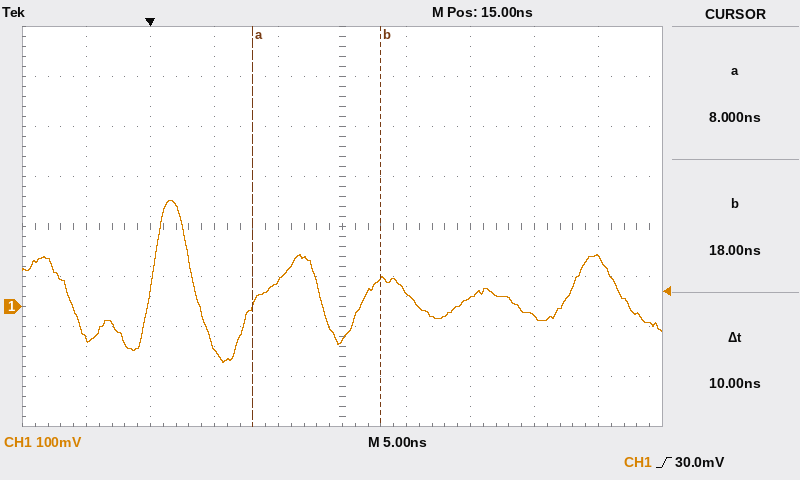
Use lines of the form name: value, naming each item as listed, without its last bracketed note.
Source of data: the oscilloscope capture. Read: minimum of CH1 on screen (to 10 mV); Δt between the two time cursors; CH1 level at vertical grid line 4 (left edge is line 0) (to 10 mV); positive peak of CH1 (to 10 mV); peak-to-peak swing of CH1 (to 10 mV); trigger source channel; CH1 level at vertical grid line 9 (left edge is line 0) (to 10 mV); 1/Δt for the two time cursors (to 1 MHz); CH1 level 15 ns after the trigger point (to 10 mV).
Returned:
minimum of CH1 on screen: -110 mV
Δt between the two time cursors: 10 ns
CH1 level at vertical grid line 4 (left edge is line 0): 50 mV
positive peak of CH1: 210 mV
peak-to-peak swing of CH1: 320 mV
trigger source channel: CH1
CH1 level at vertical grid line 9 (left edge is line 0): 100 mV
1/Δt for the two time cursors: 100 MHz
CH1 level 15 ns after the trigger point: -70 mV
